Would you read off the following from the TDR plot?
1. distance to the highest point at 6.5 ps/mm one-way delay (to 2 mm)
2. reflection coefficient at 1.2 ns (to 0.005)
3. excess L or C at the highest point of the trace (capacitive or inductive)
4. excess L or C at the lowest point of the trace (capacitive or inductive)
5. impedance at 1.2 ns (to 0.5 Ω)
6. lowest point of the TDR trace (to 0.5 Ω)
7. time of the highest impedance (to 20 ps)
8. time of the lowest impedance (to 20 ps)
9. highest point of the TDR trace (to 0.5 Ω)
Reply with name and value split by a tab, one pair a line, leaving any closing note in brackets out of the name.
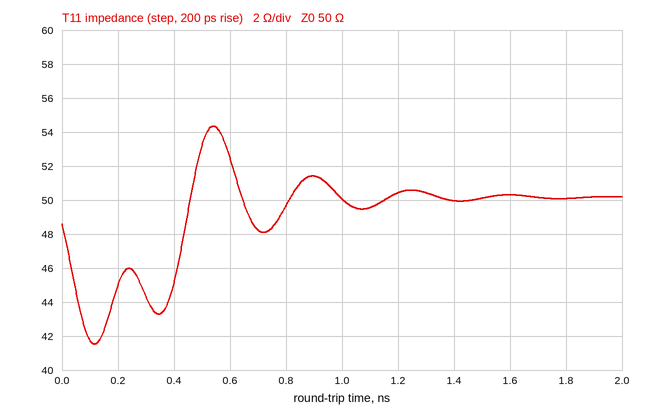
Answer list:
distance to the highest point at 6.5 ps/mm one-way delay	42 mm
reflection coefficient at 1.2 ns	+0.005
excess L or C at the highest point of the trace	inductive
excess L or C at the lowest point of the trace	capacitive
impedance at 1.2 ns	50.5 Ω
lowest point of the TDR trace	41.5 Ω
time of the highest impedance	540 ps
time of the lowest impedance	120 ps
highest point of the TDR trace	54.5 Ω
